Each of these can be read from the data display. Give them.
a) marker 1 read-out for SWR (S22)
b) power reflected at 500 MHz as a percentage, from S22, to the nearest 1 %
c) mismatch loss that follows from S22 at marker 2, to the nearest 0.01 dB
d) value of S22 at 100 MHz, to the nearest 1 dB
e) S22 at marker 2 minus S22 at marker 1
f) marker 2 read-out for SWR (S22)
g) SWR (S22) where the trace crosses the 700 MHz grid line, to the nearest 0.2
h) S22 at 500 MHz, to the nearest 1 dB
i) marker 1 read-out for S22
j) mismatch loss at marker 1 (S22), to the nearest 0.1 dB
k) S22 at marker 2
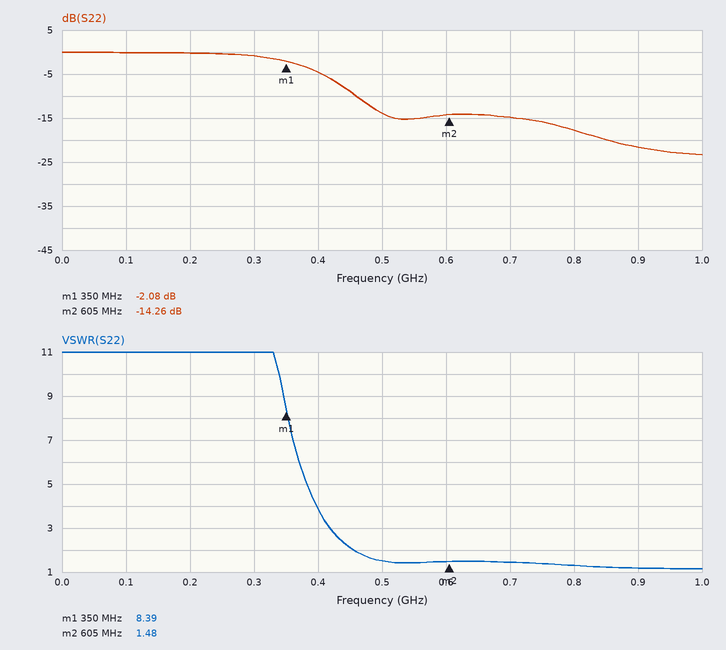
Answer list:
8.39
4 %
0.17 dB
0 dB
-12.18 dB
1.48
1.4
-14 dB
-2.08 dB
4.2 dB
-14.26 dB
